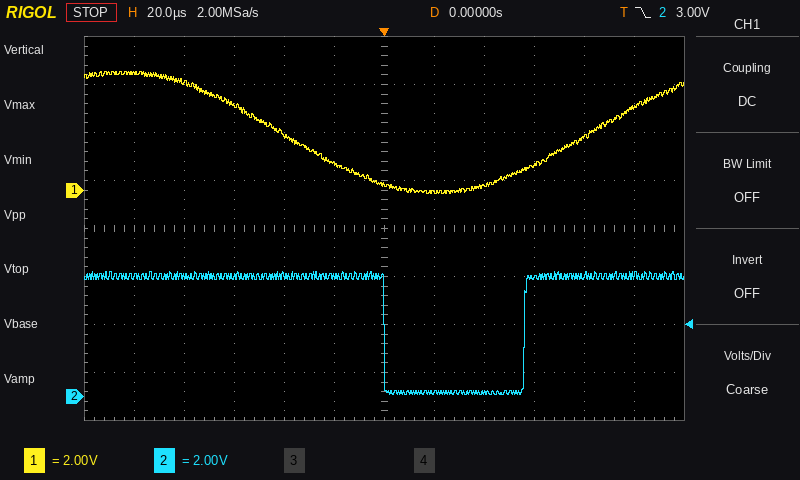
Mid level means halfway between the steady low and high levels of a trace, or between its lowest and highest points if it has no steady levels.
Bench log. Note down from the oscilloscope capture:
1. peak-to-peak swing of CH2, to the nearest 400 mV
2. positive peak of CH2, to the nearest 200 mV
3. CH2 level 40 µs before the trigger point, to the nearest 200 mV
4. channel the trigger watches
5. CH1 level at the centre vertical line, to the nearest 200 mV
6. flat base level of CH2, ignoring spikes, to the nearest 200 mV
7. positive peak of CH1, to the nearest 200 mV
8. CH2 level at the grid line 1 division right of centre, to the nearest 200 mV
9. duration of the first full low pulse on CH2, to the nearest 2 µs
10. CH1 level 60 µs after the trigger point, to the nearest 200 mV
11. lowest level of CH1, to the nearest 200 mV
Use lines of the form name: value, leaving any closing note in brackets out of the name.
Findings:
peak-to-peak swing of CH2, to the nearest 400 mV: 5.2 V
positive peak of CH2, to the nearest 200 mV: 5.2 V
CH2 level 40 µs before the trigger point, to the nearest 200 mV: 5.0 V
channel the trigger watches: CH2
CH1 level at the centre vertical line, to the nearest 200 mV: 200 mV
flat base level of CH2, ignoring spikes, to the nearest 200 mV: 200 mV
positive peak of CH1, to the nearest 200 mV: 5.0 V
CH2 level at the grid line 1 division right of centre, to the nearest 200 mV: 200 mV
duration of the first full low pulse on CH2, to the nearest 2 µs: 56 µs
CH1 level 60 µs after the trigger point, to the nearest 200 mV: 1.0 V
lowest level of CH1, to the nearest 200 mV: -200 mV
